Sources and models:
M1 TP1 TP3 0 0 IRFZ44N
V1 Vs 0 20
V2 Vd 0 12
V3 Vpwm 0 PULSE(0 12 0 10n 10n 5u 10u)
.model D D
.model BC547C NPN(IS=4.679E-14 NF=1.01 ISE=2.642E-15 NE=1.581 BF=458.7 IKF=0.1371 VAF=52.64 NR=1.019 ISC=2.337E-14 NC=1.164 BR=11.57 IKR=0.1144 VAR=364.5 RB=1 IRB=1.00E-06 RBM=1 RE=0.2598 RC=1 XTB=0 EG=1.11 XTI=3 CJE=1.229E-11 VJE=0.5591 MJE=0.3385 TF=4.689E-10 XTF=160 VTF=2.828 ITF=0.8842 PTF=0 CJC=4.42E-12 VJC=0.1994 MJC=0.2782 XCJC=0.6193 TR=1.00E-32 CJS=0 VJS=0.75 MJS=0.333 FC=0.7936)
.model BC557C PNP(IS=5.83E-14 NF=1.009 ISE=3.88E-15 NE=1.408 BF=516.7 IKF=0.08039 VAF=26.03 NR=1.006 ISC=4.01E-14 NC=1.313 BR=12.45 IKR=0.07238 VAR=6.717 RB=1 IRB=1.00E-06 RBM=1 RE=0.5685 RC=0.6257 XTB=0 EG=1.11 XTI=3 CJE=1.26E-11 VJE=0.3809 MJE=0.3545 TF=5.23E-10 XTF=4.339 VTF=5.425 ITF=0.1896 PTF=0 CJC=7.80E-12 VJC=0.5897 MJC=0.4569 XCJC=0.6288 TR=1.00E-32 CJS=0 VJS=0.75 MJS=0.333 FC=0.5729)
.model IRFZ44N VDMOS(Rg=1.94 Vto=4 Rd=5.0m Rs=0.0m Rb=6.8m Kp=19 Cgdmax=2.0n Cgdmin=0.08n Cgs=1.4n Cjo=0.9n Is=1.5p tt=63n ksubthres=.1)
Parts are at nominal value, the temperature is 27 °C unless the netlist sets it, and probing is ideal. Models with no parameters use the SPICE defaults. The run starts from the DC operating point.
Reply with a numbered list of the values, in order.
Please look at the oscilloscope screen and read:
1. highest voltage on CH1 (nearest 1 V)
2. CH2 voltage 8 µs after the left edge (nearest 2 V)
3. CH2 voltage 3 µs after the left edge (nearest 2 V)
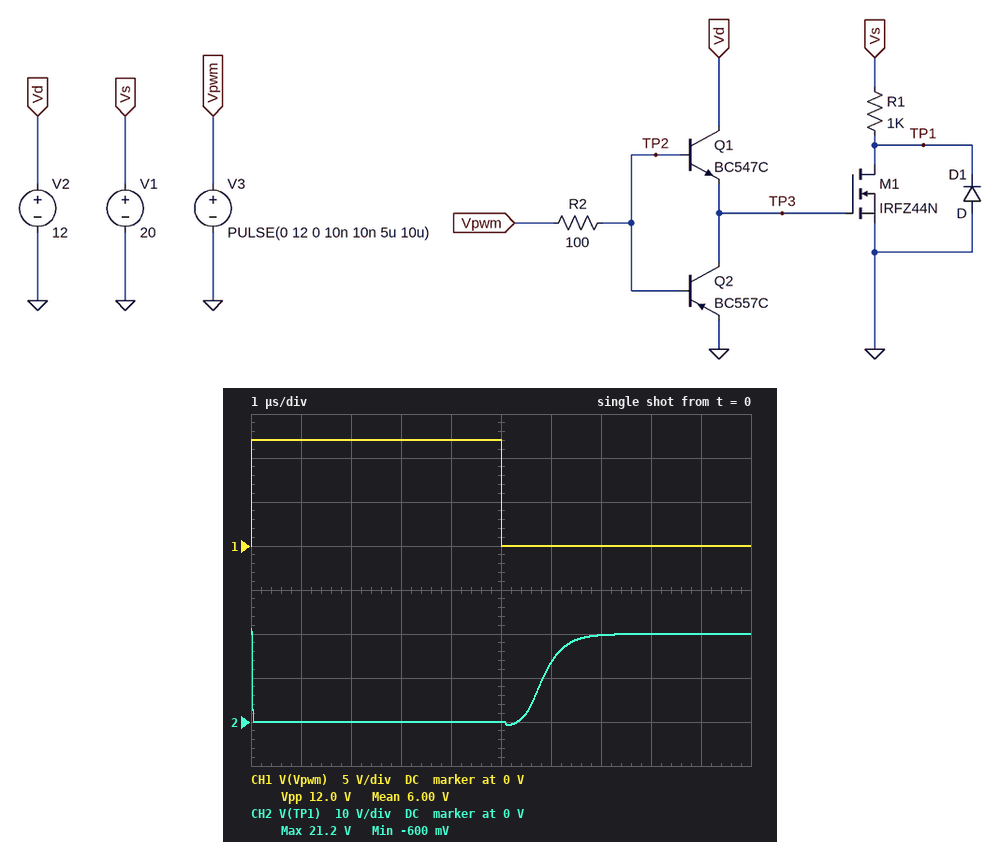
1. 12 V
2. 20 V
3. 0 V
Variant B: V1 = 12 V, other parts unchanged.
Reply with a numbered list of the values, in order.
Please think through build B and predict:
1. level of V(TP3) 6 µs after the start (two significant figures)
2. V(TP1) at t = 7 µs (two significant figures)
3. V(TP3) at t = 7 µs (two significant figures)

1. 670 mV
2. 11 V
3. 590 mV
